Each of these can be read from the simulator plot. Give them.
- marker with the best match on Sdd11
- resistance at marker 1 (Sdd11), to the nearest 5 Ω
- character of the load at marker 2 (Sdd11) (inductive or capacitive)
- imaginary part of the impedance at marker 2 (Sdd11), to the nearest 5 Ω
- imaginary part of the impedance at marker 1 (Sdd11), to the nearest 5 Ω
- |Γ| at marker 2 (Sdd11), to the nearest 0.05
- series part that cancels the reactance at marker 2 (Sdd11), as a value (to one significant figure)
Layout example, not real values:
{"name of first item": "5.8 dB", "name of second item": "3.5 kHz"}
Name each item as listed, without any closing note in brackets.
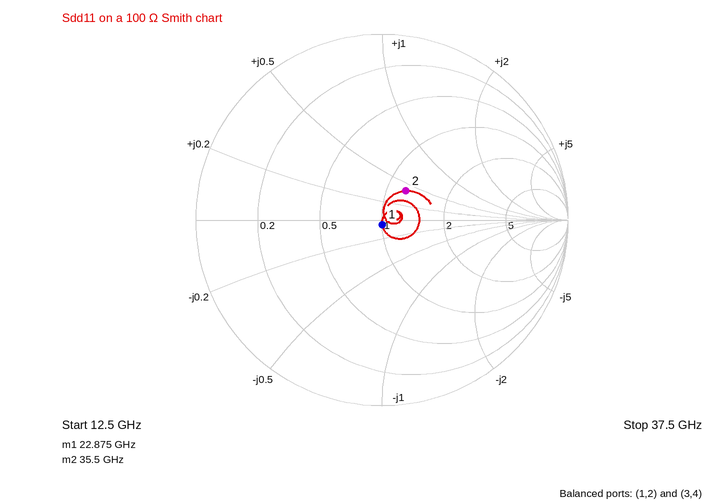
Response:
{"marker with the best match on Sdd11": "marker 1", "resistance at marker 1 (Sdd11), to the nearest 5 Ω": "100 Ω", "character of the load at marker 2 (Sdd11)": "inductive", "imaginary part of the impedance at marker 2 (Sdd11), to the nearest 5 Ω": "+40 Ω", "imaginary part of the impedance at marker 1 (Sdd11), to the nearest 5 Ω": "-5 Ω", "|Γ| at marker 2 (Sdd11), to the nearest 0.05": "0.20", "series part that cancels the reactance at marker 2 (Sdd11), as a value": "100 fF"}
